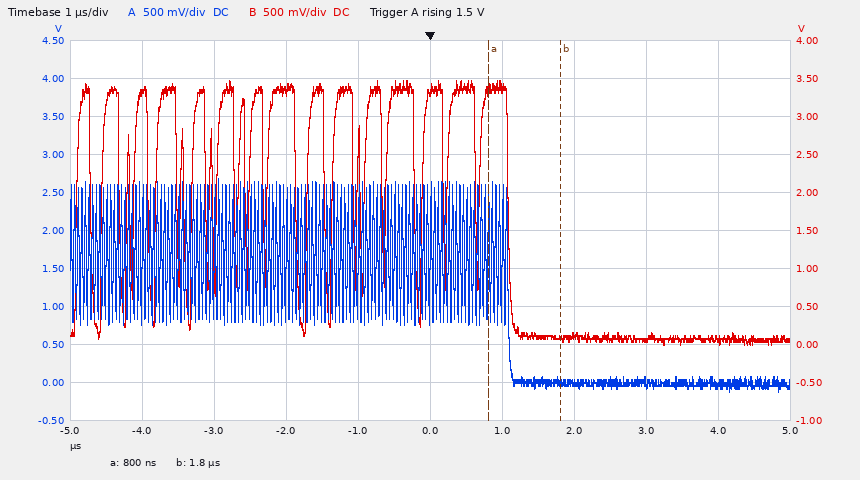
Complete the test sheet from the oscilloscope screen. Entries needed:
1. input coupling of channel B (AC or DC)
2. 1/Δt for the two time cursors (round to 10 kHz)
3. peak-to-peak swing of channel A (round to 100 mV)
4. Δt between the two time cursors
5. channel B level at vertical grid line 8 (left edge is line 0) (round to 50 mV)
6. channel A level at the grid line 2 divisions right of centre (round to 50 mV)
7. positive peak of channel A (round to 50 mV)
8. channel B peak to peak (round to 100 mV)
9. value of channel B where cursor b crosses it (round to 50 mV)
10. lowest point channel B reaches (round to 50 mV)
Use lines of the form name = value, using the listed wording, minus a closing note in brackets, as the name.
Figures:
input coupling of channel B = DC
1/Δt for the two time cursors = 1.00 MHz
peak-to-peak swing of channel A = 2.80 V
Δt between the two time cursors = 1.0 µs
channel B level at vertical grid line 8 (left edge is line 0) = 100 mV
channel A level at the grid line 2 divisions right of centre = 0 mV
positive peak of channel A = 2.70 V
channel B peak to peak = 3.50 V
value of channel B where cursor b crosses it = 100 mV
lowest point channel B reaches = 0 mV
